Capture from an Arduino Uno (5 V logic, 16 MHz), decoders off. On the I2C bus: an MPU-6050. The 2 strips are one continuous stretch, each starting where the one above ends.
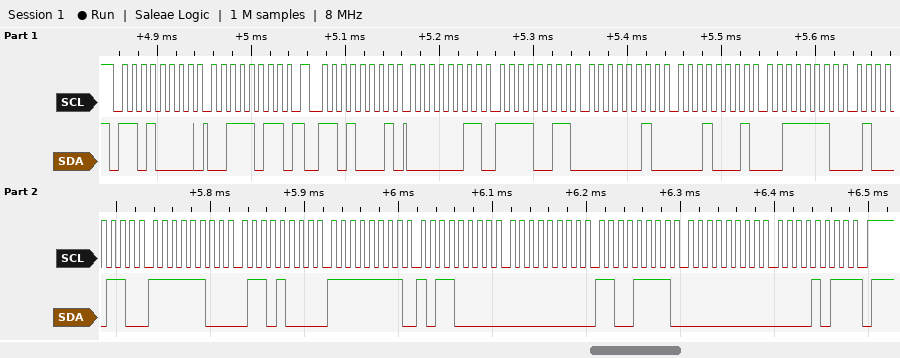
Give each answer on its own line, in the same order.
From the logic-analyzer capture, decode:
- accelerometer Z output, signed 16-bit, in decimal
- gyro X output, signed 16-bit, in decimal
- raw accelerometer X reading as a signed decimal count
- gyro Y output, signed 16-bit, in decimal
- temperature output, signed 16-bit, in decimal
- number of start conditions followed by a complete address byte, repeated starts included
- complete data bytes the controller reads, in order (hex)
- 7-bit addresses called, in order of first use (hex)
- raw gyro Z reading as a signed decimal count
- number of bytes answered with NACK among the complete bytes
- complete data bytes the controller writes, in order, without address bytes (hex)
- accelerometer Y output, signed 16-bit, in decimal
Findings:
15942
-80
1011
207
-920
2
03 F3 02 11 3E 46 FC 68 FF B0 00 CF 00 0B
0x68
11
1
3B
529
